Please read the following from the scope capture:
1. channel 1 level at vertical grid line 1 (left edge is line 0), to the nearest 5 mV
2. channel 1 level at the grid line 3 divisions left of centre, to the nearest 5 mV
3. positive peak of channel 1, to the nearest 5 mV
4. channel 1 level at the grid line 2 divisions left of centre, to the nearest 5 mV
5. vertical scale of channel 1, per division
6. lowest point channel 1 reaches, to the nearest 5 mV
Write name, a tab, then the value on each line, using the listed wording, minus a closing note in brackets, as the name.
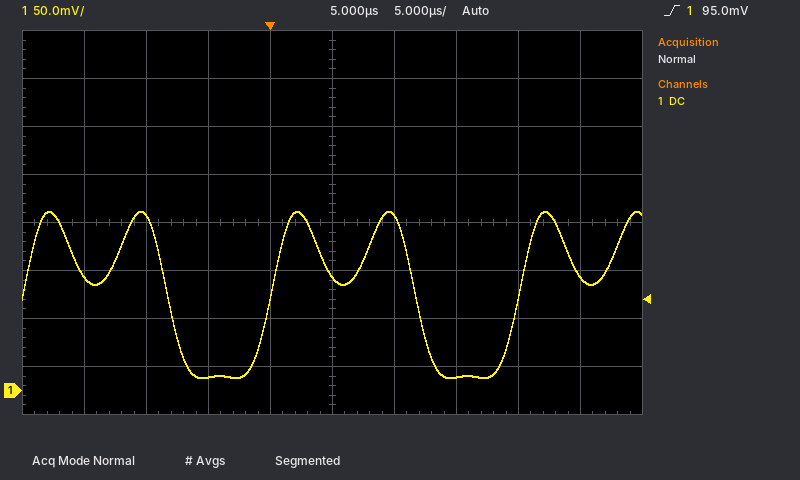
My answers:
channel 1 level at vertical grid line 1 (left edge is line 0), to the nearest 5 mV	120 mV
channel 1 level at the grid line 3 divisions left of centre, to the nearest 5 mV	180 mV
positive peak of channel 1, to the nearest 5 mV	185 mV
channel 1 level at the grid line 2 divisions left of centre, to the nearest 5 mV	15 mV
vertical scale of channel 1, per division	50 mV
lowest point channel 1 reaches, to the nearest 5 mV	15 mV
